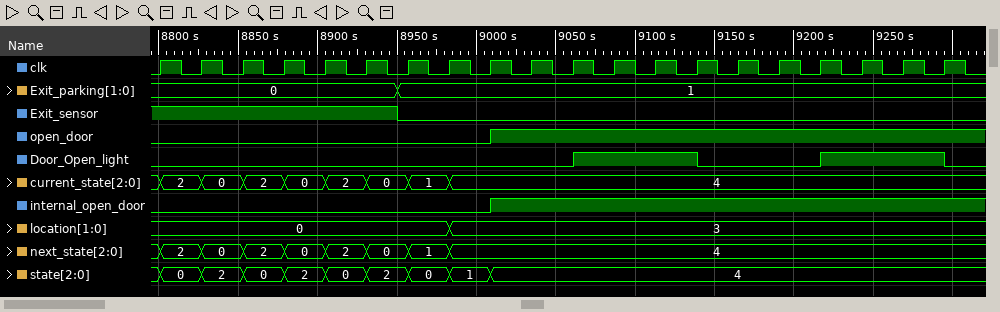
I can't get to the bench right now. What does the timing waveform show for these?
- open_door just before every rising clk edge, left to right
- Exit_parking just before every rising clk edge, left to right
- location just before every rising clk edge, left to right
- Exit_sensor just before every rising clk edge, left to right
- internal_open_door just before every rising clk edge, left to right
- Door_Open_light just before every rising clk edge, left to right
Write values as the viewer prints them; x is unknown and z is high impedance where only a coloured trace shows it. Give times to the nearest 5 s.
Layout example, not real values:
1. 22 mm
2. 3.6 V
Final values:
1. 0 0 0 0 0 0 0 0 0 1 1 1 1 1 1 1 1 1 1 1
2. 0, 0, 0, 0, 0, 0, 1, 1, 1, 1, 1, 1, 1, 1, 1, 1, 1, 1, 1, 1
3. 0, 0, 0, 0, 0, 0, 0, 0, 3, 3, 3, 3, 3, 3, 3, 3, 3, 3, 3, 3
4. 1 1 1 1 1 1 0 0 0 0 0 0 0 0 0 0 0 0 0 0
5. 0 0 0 0 0 0 0 0 0 1 1 1 1 1 1 1 1 1 1 1
6. 0 0 0 0 0 0 0 0 0 0 0 1 1 1 0 0 0 1 1 1
